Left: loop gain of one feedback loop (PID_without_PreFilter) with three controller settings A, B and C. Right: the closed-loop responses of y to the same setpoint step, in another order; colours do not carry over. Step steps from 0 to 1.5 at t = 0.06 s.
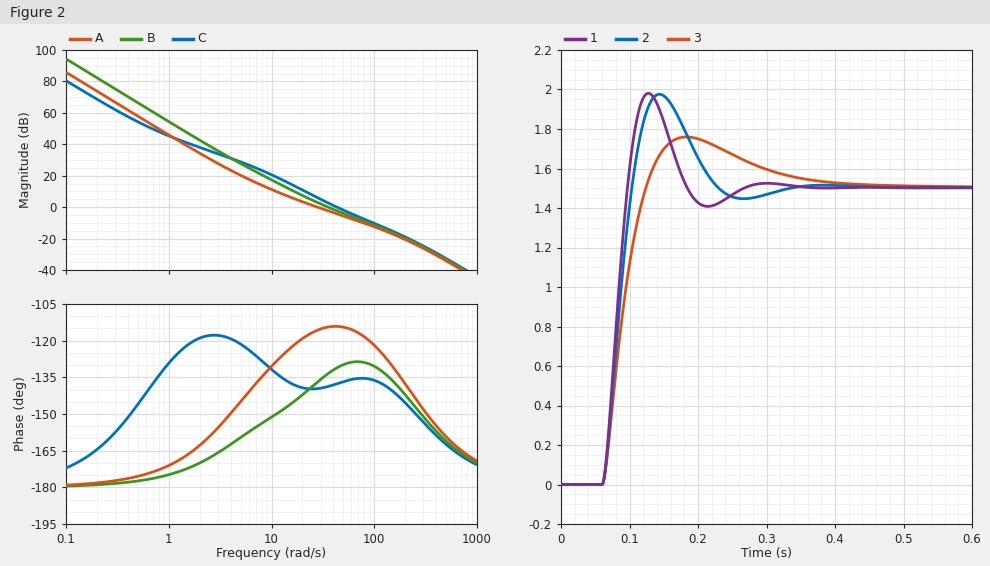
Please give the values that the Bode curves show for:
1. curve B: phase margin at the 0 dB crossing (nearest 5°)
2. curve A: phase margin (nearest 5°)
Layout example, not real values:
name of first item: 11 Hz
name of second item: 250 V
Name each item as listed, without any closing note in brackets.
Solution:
curve B: phase margin at the 0 dB crossing: 45°
curve A: phase margin: 65°
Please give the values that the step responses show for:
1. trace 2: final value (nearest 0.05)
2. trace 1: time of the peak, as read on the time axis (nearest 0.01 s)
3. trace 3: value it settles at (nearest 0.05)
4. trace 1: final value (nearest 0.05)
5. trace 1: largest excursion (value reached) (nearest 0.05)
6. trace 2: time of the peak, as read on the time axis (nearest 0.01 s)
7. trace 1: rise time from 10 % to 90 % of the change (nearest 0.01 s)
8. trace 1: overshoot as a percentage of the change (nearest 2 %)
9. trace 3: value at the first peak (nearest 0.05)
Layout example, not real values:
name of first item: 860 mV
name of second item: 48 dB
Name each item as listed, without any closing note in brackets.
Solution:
trace 2: final value: 1.50
trace 1: time of the peak, as read on the time axis: 0.13 s
trace 3: value it settles at: 1.50
trace 1: final value: 1.50
trace 1: largest excursion (value reached): 2.00
trace 2: time of the peak, as read on the time axis: 0.14 s
trace 1: rise time from 10 % to 90 % of the change: 0.03 s
trace 1: overshoot as a percentage of the change: 32 %
trace 3: value at the first peak: 1.75
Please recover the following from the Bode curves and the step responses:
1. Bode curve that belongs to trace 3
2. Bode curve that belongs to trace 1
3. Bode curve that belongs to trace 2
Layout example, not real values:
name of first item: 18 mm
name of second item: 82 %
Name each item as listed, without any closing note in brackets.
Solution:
Bode curve that belongs to trace 3: A
Bode curve that belongs to trace 1: C
Bode curve that belongs to trace 2: B
